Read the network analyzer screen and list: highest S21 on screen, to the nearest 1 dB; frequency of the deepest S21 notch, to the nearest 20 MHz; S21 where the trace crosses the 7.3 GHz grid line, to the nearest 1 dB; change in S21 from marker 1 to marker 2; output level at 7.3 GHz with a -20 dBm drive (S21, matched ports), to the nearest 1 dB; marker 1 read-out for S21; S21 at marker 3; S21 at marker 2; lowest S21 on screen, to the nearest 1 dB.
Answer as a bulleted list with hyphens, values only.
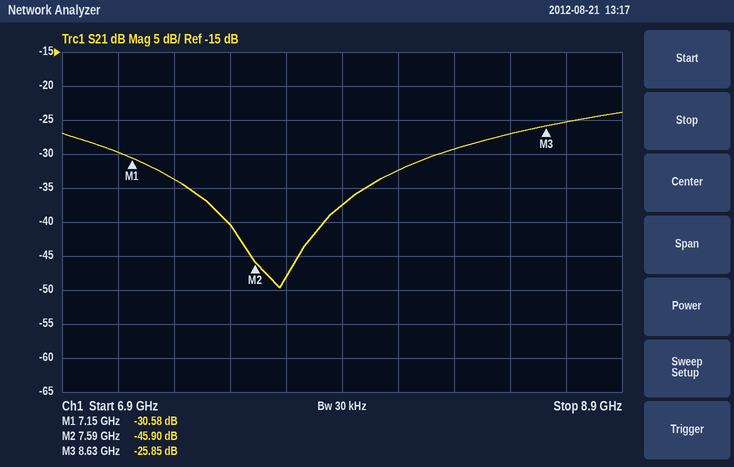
- -24 dB
- 7.68 GHz
- -34 dB
- -15.32 dB
- -54 dBm
- -30.58 dB
- -25.85 dB
- -45.90 dB
- -50 dB
